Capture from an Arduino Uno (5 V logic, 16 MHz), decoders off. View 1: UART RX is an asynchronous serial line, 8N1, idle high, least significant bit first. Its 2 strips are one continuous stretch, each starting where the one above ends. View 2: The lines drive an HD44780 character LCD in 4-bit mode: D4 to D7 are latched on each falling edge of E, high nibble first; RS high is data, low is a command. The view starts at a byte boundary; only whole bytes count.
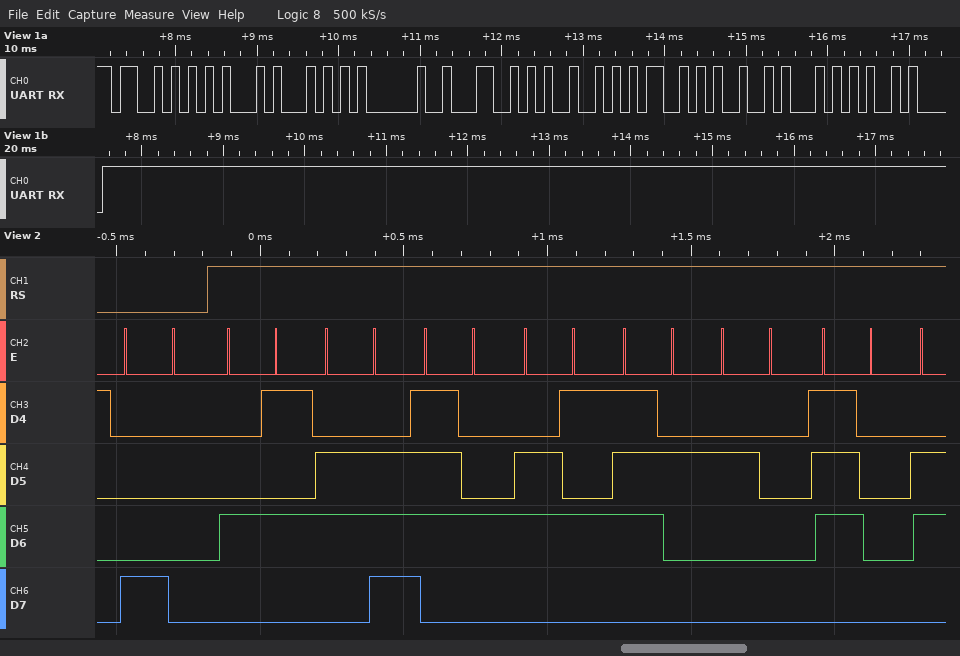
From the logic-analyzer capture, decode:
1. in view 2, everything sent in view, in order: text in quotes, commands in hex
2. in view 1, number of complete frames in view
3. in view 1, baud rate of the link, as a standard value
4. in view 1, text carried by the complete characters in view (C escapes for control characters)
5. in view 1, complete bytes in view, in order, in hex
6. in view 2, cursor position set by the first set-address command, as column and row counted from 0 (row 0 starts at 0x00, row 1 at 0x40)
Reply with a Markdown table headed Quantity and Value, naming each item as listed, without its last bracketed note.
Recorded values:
| Quantity | Value |
|---|---|
| in view 2, everything sent in view, in order: text in quotes, commands in hex | 0x80 "Enter p" |
| in view 1, number of complete frames in view | 10 |
| in view 1, baud rate of the link, as a standard value | 9600 baud |
| in view 1, text carried by the complete characters in view | "SET LIMIT\n" |
| in view 1, complete bytes in view, in order, in hex | 0x53 0x45 0x54 0x20 0x4C 0x49 0x4D 0x49 0x54 0x0A |
| in view 2, cursor position set by the first set-address command, as column and row counted from 0 | column 0, row 0 |
